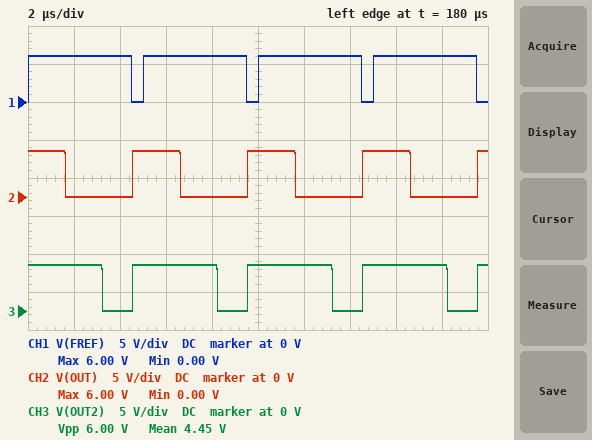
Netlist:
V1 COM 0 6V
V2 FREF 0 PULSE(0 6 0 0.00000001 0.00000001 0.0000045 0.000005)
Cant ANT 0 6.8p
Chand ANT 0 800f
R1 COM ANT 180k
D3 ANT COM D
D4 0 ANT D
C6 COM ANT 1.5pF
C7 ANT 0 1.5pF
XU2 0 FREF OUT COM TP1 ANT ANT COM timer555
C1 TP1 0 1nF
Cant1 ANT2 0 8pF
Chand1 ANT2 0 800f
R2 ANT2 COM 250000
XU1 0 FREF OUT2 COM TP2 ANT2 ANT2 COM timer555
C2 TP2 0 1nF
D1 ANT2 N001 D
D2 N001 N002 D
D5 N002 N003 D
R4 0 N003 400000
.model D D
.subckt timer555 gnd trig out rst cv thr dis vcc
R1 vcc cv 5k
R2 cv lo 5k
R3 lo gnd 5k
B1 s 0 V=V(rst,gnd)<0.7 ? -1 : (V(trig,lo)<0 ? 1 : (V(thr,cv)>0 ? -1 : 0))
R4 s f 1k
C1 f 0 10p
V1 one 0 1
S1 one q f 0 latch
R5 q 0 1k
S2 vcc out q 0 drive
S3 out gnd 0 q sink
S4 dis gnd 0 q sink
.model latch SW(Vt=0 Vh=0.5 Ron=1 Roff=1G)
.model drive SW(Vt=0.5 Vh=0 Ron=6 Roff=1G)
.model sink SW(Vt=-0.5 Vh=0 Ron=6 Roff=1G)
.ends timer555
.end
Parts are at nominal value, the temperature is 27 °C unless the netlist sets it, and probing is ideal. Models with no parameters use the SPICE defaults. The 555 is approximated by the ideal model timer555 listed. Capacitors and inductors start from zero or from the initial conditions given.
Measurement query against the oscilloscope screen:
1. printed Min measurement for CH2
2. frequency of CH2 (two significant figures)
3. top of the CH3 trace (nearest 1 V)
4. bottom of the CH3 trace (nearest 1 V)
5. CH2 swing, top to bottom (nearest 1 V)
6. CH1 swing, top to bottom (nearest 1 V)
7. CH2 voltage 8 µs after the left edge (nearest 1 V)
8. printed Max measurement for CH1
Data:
0.00 V
200 kHz
6 V
0 V
6 V
6 V
0 V
6.00 V
